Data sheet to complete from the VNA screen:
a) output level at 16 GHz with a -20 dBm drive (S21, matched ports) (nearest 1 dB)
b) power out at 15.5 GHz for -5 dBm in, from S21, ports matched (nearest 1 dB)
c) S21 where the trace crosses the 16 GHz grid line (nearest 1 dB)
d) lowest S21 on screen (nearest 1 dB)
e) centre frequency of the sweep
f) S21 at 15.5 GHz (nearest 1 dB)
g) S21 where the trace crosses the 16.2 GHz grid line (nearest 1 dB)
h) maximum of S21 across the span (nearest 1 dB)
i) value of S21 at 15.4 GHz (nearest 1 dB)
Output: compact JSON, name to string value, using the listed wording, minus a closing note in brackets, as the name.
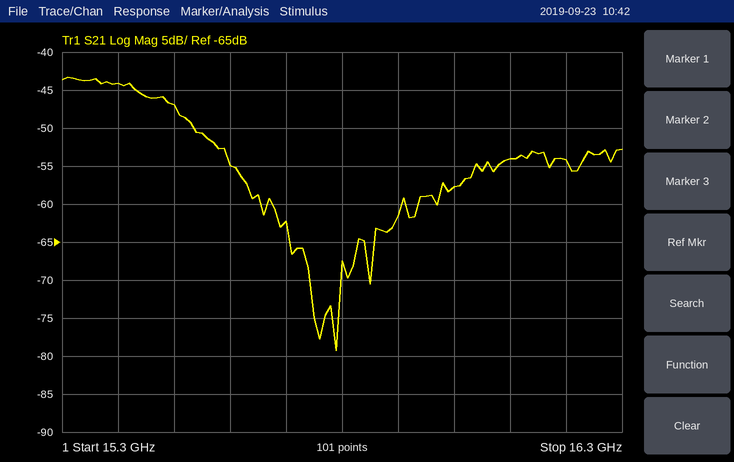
{"output level at 16 GHz with a -20 dBm drive (S21, matched ports)": "-78 dBm", "power out at 15.5 GHz for -5 dBm in, from S21, ports matched": "-52 dBm", "S21 where the trace crosses the 16 GHz grid line": "-58 dB", "lowest S21 on screen": "-79 dB", "centre frequency of the sweep": "15.8 GHz", "S21 at 15.5 GHz": "-47 dB", "S21 where the trace crosses the 16.2 GHz grid line": "-54 dB", "maximum of S21 across the span": "-43 dB", "value of S21 at 15.4 GHz": "-44 dB"}
